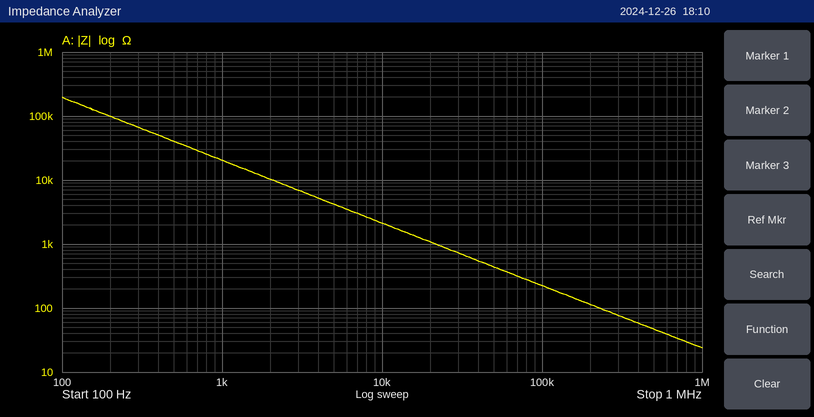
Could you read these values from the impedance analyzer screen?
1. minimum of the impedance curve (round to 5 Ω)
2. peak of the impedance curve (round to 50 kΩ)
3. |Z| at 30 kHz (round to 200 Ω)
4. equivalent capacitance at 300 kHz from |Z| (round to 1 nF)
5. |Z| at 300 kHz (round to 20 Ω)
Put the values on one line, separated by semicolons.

25 Ω; 200 kΩ; 800 Ω; 7 nF; 80 Ω
